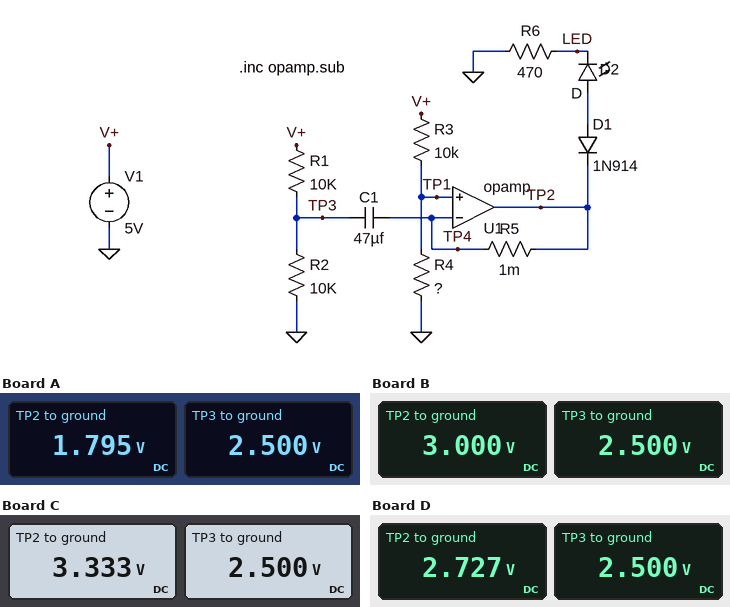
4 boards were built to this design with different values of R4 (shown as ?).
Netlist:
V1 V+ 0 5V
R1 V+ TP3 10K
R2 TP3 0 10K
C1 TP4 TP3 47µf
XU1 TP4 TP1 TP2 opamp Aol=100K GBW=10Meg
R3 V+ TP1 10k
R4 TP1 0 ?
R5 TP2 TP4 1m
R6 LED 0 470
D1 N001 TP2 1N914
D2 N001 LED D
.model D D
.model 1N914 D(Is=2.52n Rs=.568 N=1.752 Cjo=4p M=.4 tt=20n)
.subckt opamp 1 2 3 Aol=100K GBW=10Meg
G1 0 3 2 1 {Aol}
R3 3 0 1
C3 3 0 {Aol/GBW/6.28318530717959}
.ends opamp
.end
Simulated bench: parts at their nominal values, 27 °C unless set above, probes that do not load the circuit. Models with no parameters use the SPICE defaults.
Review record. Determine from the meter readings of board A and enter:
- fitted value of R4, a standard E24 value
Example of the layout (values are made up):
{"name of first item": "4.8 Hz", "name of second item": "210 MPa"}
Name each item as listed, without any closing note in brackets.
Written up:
{"fitted value of R4, a standard E24 value": "5.6 kΩ"}
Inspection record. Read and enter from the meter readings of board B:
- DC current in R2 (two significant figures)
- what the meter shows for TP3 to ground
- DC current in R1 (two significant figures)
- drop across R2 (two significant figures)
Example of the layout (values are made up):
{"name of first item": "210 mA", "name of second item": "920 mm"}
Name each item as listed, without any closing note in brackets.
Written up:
{"DC current in R2": "250 µA", "what the meter shows for TP3 to ground": "2.500 V", "DC current in R1": "250 µA", "drop across R2": "2.5 V"}
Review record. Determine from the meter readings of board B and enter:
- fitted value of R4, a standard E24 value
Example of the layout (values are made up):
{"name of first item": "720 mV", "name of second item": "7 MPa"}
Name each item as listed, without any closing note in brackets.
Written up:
{"fitted value of R4, a standard E24 value": "15 kΩ"}
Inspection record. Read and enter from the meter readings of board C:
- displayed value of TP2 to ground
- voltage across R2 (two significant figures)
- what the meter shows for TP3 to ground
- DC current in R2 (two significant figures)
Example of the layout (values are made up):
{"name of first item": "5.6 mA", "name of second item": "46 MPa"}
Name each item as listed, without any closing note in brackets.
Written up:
{"displayed value of TP2 to ground": "3.333 V", "voltage across R2": "2.5 V", "what the meter shows for TP3 to ground": "2.500 V", "DC current in R2": "250 µA"}
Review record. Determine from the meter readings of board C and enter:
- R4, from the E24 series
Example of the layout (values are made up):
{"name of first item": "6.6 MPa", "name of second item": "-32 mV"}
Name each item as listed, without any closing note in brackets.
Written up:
{"R4, from the E24 series": "20 kΩ"}
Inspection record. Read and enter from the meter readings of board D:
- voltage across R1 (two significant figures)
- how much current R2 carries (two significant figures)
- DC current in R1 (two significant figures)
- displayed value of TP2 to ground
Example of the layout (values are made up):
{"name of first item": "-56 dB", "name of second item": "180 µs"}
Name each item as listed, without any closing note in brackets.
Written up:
{"voltage across R1": "2.5 V", "how much current R2 carries": "250 µA", "DC current in R1": "250 µA", "displayed value of TP2 to ground": "2.727 V"}
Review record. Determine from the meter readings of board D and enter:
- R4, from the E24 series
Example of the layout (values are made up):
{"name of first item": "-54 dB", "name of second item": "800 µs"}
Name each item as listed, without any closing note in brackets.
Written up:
{"R4, from the E24 series": "12 kΩ"}
